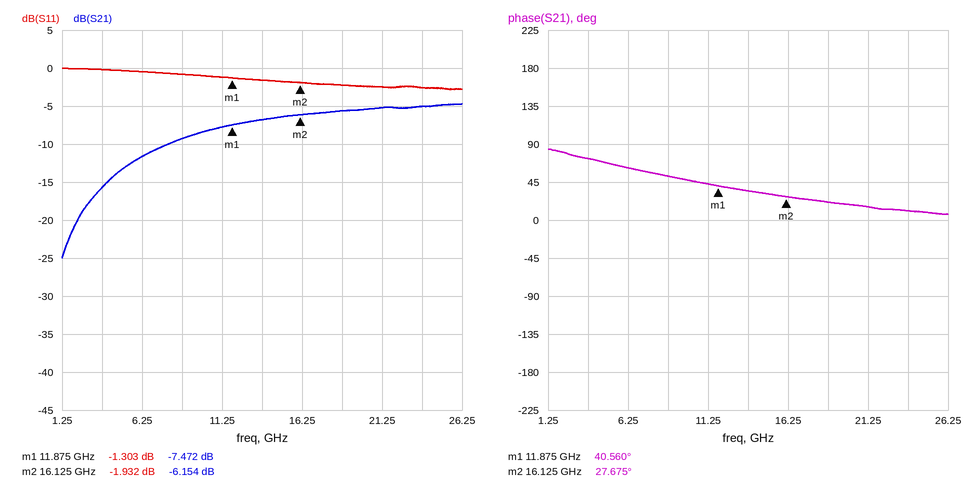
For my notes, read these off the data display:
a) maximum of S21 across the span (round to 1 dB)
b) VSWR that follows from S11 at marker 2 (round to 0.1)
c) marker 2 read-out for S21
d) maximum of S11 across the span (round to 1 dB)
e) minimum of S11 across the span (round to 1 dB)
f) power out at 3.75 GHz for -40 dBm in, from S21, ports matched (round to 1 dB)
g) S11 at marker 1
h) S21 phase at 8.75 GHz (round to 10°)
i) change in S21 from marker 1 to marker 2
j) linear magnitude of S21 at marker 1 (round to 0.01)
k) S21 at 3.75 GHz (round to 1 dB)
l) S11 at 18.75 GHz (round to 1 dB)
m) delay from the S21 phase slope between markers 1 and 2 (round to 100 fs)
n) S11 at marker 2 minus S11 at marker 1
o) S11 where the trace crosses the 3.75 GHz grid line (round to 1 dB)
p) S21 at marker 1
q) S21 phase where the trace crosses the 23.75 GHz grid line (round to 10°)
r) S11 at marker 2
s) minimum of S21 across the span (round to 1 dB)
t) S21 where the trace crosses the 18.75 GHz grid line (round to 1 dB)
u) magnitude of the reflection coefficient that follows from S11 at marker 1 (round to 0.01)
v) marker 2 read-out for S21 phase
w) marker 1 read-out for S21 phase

-5 dB
9.0
-6.154 dB
0 dB
-3 dB
-56 dBm
-1.303 dB
50°
1.318 dB
0.42
-16 dB
-2 dB
8.4 ps
-0.629 dB
0 dB
-7.472 dB
10°
-1.932 dB
-25 dB
-6 dB
0.86
27.675°
40.560°
